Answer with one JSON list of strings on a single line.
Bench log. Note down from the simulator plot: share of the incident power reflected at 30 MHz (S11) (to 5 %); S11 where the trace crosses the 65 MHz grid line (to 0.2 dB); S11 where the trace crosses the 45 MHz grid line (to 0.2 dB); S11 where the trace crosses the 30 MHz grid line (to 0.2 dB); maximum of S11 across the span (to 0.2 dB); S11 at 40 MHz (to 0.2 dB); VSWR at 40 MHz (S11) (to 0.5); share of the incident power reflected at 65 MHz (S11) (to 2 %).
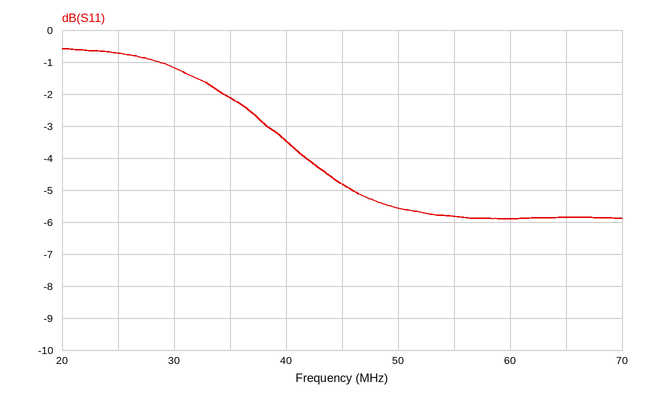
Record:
["75 %", "-5.8 dB", "-4.8 dB", "-1.2 dB", "-0.6 dB", "-3.4 dB", "5.0", "26 %"]
